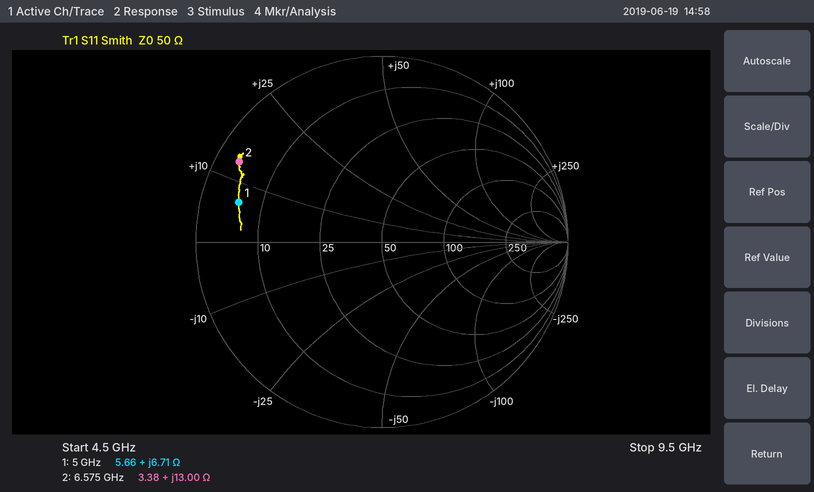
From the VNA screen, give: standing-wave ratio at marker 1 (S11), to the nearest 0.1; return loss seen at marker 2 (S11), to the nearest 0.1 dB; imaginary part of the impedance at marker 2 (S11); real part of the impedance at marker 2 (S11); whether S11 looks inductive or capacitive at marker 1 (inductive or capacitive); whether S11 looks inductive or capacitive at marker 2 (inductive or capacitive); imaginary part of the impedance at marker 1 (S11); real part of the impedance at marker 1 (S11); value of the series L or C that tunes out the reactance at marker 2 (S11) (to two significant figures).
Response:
9.0
1.1 dB
+13.00 Ω
3.38 Ω
inductive
inductive
+6.71 Ω
5.66 Ω
1.9 pF
